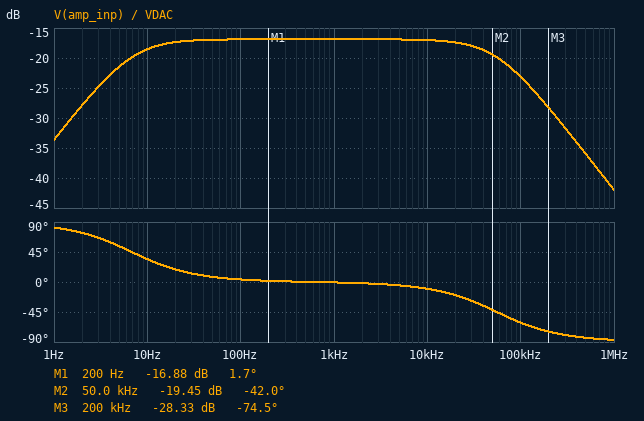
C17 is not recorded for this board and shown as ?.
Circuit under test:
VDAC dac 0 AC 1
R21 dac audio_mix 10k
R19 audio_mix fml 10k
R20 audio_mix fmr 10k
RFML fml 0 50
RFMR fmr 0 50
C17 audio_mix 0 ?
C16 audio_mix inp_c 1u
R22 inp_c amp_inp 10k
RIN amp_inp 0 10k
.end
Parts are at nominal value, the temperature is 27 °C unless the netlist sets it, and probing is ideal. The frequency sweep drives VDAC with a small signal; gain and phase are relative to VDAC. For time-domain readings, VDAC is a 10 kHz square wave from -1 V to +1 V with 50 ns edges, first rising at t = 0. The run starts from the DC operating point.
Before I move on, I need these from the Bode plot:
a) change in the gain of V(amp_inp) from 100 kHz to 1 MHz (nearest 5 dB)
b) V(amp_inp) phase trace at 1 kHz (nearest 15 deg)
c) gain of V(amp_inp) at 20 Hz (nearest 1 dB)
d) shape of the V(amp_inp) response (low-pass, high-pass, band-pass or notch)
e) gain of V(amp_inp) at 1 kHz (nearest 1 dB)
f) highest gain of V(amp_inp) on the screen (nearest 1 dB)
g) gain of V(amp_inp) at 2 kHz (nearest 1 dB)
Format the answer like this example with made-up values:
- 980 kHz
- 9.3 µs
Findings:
- -20 dB
- 0 deg
- -17 dB
- band-pass
- -17 dB
- -17 dB
- -17 dB
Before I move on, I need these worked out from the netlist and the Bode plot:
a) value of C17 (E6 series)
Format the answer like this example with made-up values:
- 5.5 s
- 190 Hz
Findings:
- 1 nF
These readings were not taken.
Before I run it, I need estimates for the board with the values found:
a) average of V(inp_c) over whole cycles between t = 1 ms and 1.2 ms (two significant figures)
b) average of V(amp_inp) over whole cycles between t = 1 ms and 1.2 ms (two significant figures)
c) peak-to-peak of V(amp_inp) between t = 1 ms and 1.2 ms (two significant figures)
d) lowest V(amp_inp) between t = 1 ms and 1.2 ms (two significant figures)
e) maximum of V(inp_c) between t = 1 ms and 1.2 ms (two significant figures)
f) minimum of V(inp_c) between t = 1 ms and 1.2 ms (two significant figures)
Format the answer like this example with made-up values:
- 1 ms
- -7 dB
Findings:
- 270 mV
- 140 mV
- 290 mV
- -7.2 mV
- 560 mV
- -14 mV
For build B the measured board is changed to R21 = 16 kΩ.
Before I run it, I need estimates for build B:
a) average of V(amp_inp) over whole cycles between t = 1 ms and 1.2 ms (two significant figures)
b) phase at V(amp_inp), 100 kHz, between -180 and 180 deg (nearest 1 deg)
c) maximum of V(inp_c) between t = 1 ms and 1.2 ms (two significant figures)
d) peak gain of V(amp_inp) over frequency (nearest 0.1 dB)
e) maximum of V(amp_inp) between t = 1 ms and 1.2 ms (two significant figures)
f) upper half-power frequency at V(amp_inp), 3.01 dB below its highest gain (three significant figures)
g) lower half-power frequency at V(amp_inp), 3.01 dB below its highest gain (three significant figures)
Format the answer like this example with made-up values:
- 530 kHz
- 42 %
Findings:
- 96 mV
- -64 deg
- 390 mV
- -20.0 dB
- 200 mV
- 49.6 kHz
- 6.68 Hz
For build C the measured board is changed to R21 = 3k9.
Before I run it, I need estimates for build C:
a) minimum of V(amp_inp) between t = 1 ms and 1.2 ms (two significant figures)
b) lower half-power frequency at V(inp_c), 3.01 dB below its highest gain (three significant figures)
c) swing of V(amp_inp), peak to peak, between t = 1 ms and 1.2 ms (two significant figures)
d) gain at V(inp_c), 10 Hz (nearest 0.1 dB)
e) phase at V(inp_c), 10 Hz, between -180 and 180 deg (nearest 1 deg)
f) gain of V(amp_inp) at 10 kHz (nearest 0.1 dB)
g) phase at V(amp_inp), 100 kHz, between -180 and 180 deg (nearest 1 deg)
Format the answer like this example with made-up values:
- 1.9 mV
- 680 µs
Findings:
- -13 mV
- 7.17 Hz
- 510 mV
- -7.7 dB
- 36 deg
- -12.0 dB
- -51 deg
